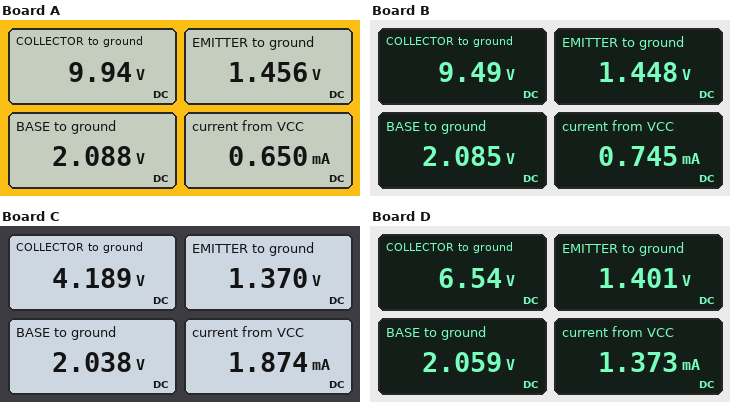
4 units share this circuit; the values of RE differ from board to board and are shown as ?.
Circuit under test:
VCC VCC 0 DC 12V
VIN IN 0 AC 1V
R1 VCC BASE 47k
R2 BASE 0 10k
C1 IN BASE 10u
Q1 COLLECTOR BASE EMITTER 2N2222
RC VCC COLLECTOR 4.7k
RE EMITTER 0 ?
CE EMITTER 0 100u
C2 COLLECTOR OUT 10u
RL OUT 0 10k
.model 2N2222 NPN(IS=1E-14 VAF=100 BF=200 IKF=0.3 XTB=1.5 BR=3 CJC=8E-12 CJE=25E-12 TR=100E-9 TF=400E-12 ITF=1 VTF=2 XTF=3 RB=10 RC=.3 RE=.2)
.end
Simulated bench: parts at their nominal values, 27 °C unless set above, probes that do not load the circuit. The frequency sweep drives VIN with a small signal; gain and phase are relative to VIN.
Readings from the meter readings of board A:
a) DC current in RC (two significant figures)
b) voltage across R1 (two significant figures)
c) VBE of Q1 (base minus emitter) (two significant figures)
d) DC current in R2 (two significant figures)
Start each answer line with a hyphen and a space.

- 440 µA
- 9.9 V
- 630 mV
- 210 µA
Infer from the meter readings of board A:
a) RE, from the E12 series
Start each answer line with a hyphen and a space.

- 3.3 kΩ
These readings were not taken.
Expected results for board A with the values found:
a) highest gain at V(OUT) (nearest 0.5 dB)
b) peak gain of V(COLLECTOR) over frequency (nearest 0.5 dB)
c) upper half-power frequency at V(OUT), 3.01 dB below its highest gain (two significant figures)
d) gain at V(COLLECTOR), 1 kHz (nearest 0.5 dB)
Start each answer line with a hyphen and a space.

- 34.5 dB
- 34.5 dB
- 12 MHz
- 34.5 dB
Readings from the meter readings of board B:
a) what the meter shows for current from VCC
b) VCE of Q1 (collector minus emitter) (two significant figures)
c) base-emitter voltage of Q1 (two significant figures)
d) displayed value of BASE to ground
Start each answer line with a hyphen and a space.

- 0.745 mA
- 8.0 V
- 640 mV
- 2.085 V
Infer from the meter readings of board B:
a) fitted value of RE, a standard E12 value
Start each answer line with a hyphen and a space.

- 2.7 kΩ
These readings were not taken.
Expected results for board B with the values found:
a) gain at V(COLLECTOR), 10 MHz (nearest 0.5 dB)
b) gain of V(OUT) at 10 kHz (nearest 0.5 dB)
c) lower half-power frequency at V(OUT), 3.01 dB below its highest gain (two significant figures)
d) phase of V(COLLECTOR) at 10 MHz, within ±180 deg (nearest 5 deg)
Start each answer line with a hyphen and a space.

- 33.5 dB
- 36.0 dB
- 35 Hz
- 135 deg
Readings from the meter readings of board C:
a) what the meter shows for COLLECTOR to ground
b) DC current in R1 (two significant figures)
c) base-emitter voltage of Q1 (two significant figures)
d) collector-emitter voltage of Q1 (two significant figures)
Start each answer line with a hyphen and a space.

- 4.189 V
- 210 µA
- 670 mV
- 2.8 V
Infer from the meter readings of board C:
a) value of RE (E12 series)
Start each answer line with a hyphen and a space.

- 820 Ω
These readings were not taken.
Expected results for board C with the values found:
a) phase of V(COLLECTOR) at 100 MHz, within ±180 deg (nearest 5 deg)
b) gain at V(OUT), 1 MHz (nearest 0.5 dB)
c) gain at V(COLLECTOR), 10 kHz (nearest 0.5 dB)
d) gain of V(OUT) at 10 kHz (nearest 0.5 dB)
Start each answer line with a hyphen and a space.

- 75 deg
- 45.5 dB
- 45.5 dB
- 45.5 dB
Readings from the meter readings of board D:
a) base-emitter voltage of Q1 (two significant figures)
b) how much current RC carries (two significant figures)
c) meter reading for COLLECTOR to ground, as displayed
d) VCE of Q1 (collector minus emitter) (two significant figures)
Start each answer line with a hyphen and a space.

- 660 mV
- 1.2 mA
- 6.54 V
- 5.1 V
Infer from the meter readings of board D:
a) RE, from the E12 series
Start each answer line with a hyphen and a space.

- 1.2 kΩ
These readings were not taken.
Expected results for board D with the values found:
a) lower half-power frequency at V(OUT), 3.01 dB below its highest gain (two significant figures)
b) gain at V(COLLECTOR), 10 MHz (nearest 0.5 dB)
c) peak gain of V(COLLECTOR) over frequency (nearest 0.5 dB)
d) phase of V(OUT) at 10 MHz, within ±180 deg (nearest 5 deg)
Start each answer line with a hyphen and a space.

- 73 Hz
- 39.0 dB
- 42.5 dB
- 130 deg
